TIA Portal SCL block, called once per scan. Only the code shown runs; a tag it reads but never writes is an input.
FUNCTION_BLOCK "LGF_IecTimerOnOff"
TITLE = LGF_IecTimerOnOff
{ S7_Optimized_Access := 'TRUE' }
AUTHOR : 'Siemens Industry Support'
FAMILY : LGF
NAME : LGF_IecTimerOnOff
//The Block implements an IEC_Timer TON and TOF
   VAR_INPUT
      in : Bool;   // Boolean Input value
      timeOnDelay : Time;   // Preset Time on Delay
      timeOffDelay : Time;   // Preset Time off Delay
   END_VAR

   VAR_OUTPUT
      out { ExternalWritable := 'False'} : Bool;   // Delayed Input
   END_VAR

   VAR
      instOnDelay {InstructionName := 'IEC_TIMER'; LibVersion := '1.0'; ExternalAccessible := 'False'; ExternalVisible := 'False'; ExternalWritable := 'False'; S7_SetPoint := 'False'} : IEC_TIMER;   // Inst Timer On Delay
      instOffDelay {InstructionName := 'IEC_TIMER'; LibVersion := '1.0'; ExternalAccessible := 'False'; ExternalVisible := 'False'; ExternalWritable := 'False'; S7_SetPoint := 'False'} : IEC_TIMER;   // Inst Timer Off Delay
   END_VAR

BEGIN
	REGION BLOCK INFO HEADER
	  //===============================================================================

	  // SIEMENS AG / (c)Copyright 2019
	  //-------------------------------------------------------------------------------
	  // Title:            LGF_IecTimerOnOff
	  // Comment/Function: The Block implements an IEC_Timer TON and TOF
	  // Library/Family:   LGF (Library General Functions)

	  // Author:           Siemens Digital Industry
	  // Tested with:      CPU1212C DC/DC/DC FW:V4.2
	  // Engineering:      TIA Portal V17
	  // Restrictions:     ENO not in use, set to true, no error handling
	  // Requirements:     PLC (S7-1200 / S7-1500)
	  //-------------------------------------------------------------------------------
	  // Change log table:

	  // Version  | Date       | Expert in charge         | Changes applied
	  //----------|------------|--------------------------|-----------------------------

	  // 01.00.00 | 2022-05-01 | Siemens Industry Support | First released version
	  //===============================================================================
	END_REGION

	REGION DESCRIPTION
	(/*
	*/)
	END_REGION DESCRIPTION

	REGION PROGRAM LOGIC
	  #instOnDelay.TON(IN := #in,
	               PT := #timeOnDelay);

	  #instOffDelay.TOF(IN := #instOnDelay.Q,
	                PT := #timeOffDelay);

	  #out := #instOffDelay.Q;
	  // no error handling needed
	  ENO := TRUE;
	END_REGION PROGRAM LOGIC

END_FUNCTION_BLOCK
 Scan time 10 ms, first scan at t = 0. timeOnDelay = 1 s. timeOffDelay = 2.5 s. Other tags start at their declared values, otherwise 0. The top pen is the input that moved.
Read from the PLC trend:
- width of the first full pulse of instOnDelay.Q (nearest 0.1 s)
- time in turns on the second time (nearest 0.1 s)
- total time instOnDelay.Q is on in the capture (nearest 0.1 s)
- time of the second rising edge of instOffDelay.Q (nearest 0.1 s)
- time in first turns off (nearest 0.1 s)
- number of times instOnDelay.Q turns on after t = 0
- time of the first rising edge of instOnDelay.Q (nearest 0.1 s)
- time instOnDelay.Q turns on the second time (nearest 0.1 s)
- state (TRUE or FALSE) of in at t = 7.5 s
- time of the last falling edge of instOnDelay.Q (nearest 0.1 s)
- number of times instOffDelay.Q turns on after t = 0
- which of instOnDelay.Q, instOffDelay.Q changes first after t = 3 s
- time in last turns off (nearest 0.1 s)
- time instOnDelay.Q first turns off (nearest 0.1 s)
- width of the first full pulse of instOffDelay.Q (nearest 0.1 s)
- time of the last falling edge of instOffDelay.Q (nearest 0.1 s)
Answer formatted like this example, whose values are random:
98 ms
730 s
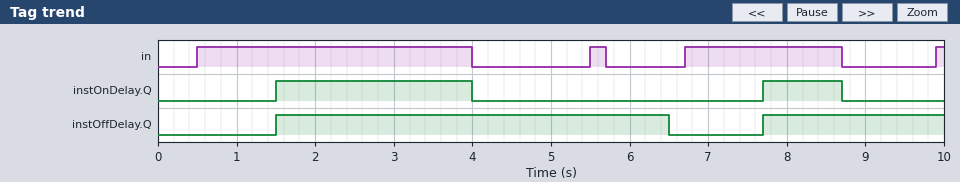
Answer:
2.5 s
5.5 s
3.5 s
7.7 s
4.0 s
2
1.5 s
7.7 s
TRUE
8.7 s
2
instOnDelay.Q
8.7 s
4.0 s
5.0 s
6.5 s
